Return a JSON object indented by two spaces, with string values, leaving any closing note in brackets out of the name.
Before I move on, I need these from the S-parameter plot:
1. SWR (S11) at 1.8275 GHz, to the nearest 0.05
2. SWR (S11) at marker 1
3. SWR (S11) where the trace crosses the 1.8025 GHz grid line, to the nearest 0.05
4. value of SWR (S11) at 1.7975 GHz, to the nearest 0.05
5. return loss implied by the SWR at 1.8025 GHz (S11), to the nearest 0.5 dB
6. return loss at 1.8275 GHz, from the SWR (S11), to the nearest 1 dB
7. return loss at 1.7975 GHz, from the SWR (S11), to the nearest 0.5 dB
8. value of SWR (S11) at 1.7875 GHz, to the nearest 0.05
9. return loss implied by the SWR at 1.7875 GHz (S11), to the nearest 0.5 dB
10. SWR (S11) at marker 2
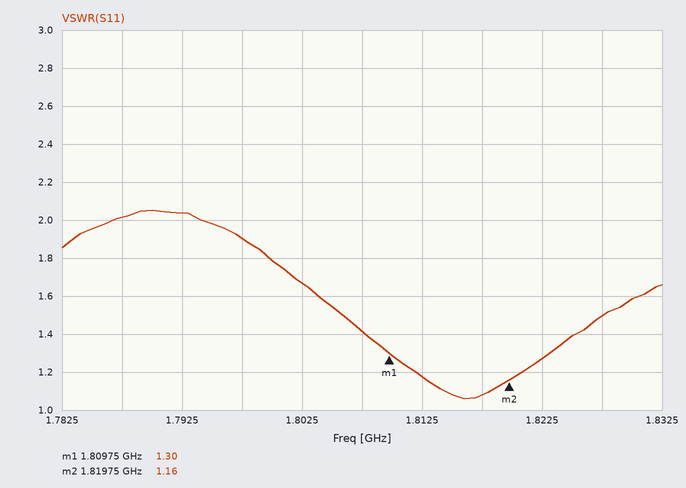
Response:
{
  "SWR (S11) at 1.8275 GHz, to the nearest 0.05": "1.50",
  "SWR (S11) at marker 1": "1.30",
  "SWR (S11) where the trace crosses the 1.8025 GHz grid line, to the nearest 0.05": "1.65",
  "value of SWR (S11) at 1.7975 GHz, to the nearest 0.05": "1.90",
  "return loss implied by the SWR at 1.8025 GHz (S11), to the nearest 0.5 dB": "12.0 dB",
  "return loss at 1.8275 GHz, from the SWR (S11), to the nearest 1 dB": "14 dB",
  "return loss at 1.7975 GHz, from the SWR (S11), to the nearest 0.5 dB": "10.0 dB",
  "value of SWR (S11) at 1.7875 GHz, to the nearest 0.05": "2.00",
  "return loss implied by the SWR at 1.7875 GHz (S11), to the nearest 0.5 dB": "9.5 dB",
  "SWR (S11) at marker 2": "1.16"
}
